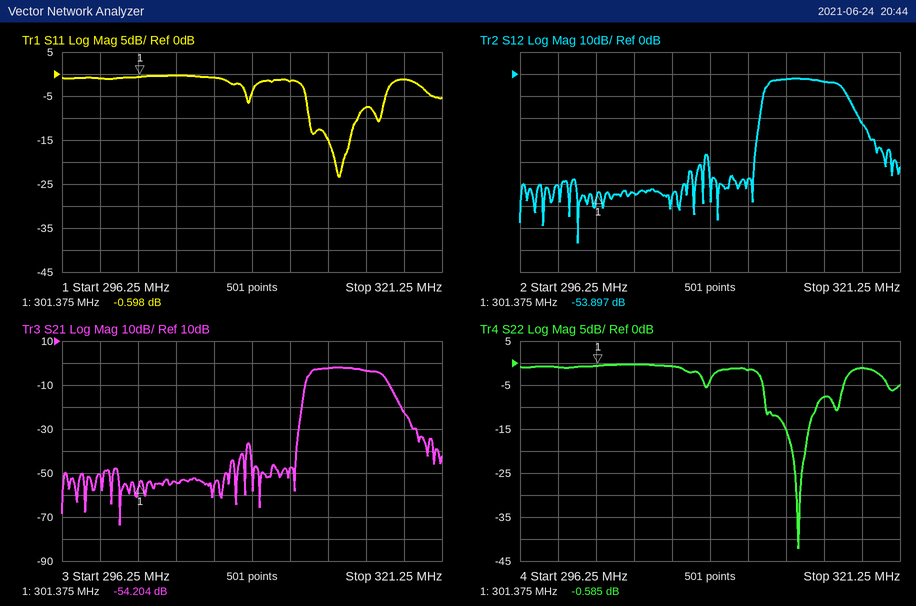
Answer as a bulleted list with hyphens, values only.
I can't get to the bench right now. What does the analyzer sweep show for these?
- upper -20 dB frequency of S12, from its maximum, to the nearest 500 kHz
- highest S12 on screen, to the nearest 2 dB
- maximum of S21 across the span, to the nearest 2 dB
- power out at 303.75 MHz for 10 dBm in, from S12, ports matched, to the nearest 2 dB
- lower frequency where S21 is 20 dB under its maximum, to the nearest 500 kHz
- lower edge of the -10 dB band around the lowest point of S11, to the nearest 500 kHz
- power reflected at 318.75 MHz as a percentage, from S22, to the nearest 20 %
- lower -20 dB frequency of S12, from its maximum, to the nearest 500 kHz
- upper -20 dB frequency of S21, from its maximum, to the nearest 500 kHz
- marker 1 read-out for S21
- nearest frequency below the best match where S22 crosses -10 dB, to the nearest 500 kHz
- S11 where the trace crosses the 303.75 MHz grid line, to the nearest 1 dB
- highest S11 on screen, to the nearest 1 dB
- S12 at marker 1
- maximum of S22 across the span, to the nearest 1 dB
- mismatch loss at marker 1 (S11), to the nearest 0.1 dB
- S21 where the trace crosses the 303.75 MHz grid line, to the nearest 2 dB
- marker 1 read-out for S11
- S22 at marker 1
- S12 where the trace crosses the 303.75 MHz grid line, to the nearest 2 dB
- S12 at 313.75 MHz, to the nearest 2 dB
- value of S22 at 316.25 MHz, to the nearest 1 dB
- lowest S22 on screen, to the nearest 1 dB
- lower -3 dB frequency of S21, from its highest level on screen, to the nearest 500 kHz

- 318.5 MHz
- -2 dB
- -2 dB
- -44 dBm
- 312.0 MHz
- 312.5 MHz
- 80 %
- 312.0 MHz
- 318.5 MHz
- -54.204 dB
- 312.5 MHz
- 0 dB
- 0 dB
- -53.897 dB
- 0 dB
- 8.9 dB
- -54 dB
- -0.598 dB
- -0.585 dB
- -54 dB
- -2 dB
- -8 dB
- -42 dB
- 312.5 MHz
